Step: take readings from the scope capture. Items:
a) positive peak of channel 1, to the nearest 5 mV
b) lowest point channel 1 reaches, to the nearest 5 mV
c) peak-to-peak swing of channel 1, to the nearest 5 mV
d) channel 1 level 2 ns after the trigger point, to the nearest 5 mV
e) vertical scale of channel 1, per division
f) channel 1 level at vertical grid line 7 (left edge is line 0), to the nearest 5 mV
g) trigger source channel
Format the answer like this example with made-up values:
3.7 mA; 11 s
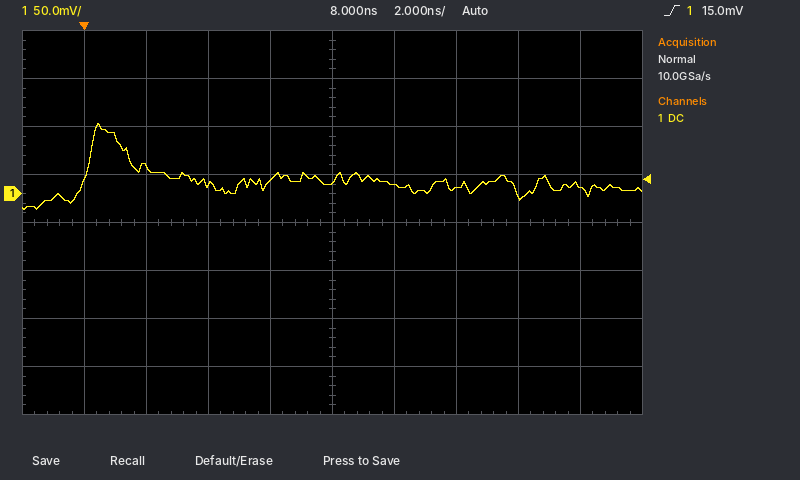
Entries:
75 mV; -15 mV; 90 mV; 30 mV; 50 mV; 5 mV; channel 1
